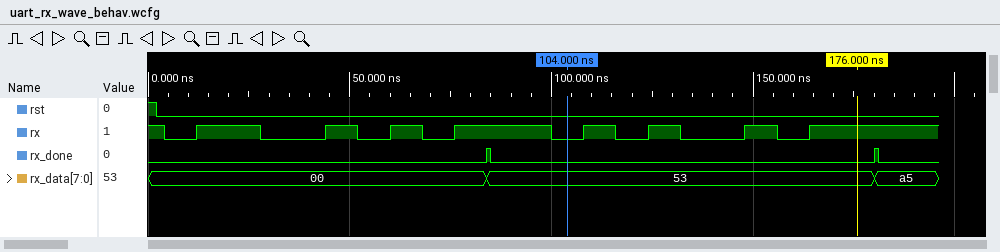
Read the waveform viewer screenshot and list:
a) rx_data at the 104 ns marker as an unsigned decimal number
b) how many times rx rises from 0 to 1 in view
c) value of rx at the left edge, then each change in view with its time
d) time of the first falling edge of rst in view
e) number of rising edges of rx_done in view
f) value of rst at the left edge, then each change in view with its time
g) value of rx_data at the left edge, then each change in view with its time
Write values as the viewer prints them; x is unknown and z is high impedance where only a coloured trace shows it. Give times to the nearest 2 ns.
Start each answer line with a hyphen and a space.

- 83
- 8
- 1, 0 at 4 ns, 1 at 12 ns, 0 at 28 ns, 1 at 44 ns, 0 at 52 ns, 1 at 60 ns, 0 at 68 ns, 1 at 76 ns, 0 at 100 ns, 1 at 108 ns, 0 at 116 ns, 1 at 124 ns, 0 at 132 ns, 1 at 148 ns, 0 at 156 ns, 1 at 164 ns
- 2 ns
- 2
- 1, 0 at 2 ns
- 00, 53 at 84 ns, a5 at 180 ns
